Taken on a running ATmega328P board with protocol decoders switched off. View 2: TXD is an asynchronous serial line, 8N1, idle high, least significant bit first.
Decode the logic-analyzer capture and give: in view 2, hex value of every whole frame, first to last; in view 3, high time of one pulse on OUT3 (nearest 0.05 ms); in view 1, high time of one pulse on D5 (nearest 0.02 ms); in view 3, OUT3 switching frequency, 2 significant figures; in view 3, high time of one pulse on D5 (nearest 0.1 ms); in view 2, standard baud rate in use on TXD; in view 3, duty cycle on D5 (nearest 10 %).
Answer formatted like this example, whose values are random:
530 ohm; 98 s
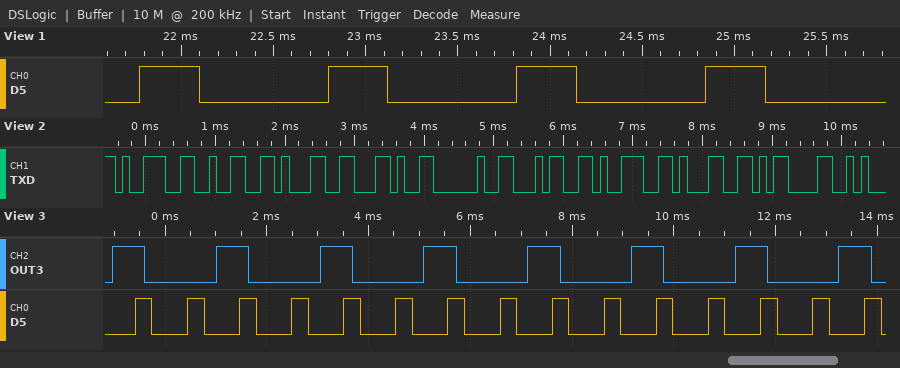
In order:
0x39 0x32 0x31 0x2C 0x20 0x34 0x39 0x31 0x0D; 0.65 ms; 0.32 ms; 490 Hz; 0.3 ms; 9600 baud; 30 %
